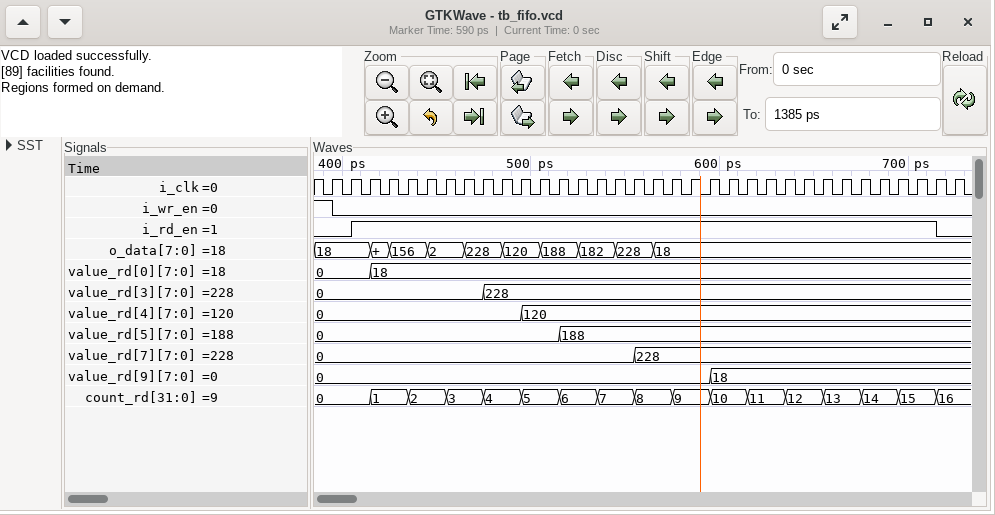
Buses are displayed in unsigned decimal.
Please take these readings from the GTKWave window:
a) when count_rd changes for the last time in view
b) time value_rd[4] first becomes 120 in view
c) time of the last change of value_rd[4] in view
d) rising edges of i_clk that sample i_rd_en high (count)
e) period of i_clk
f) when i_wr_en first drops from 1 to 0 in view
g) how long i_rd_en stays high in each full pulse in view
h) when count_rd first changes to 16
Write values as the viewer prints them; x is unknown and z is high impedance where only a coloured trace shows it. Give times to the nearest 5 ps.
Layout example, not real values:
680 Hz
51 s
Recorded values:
715 ps
495 ps
495 ps
31
10 ps
395 ps
310 ps
715 ps
